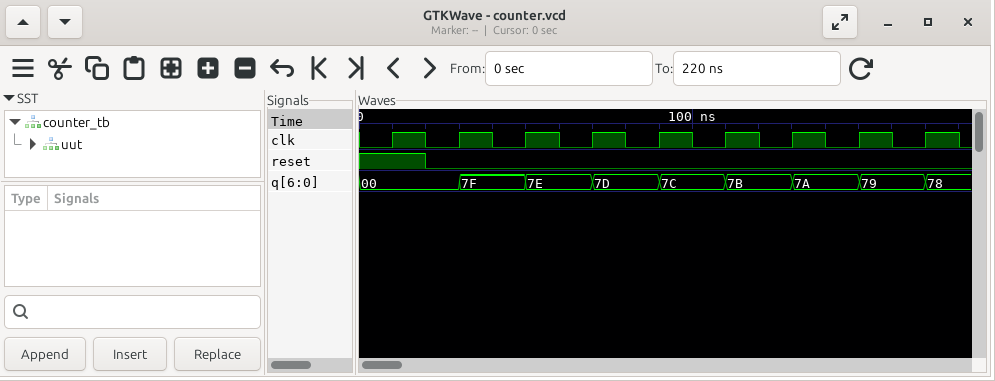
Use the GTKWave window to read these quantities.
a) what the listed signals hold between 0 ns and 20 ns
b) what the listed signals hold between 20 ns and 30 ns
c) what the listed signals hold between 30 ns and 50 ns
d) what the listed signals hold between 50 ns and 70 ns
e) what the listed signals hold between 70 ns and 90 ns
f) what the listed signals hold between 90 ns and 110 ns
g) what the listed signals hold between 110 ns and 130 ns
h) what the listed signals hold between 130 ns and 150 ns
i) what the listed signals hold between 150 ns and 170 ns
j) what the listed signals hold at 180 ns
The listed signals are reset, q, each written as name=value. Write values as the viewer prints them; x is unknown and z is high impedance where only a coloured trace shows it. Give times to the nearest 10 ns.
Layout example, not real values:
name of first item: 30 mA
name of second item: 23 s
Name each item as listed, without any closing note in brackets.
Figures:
what the listed signals hold between 0 ns and 20 ns: reset=1, q=00
what the listed signals hold between 20 ns and 30 ns: reset=0, q=00
what the listed signals hold between 30 ns and 50 ns: reset=0, q=7F
what the listed signals hold between 50 ns and 70 ns: reset=0, q=7E
what the listed signals hold between 70 ns and 90 ns: reset=0, q=7D
what the listed signals hold between 90 ns and 110 ns: reset=0, q=7C
what the listed signals hold between 110 ns and 130 ns: reset=0, q=7B
what the listed signals hold between 130 ns and 150 ns: reset=0, q=7A
what the listed signals hold between 150 ns and 170 ns: reset=0, q=79
what the listed signals hold at 180 ns: reset=0, q=78
